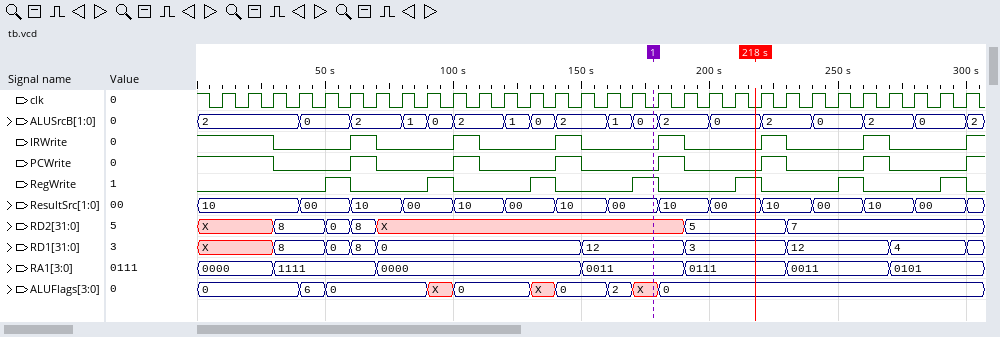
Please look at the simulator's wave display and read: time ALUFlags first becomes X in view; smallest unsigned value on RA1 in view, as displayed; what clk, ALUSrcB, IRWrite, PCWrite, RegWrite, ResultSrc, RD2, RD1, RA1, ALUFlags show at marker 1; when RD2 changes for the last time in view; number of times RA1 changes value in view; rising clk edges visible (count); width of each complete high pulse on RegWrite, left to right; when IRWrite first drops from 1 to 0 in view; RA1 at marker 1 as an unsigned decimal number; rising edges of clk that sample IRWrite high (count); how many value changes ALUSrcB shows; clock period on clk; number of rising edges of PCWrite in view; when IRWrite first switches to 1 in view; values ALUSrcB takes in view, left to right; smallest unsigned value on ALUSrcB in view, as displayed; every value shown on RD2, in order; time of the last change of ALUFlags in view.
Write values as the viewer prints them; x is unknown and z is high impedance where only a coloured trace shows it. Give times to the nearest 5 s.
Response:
90 s
0000
clk=0, ALUSrcB=0, IRWrite=0, PCWrite=0, RegWrite=1, ResultSrc=00, RD2=X, RD1=12, RA1=0011, ALUFlags=X
230 s
6
30
10 s, 10 s, 10 s, 10 s, 10 s, 10 s, 10 s
30 s
3
9
17
10 s
7
60 s
2, 0, 2, 1, 0, 2, 1, 0, 2, 1, 0, 2, 0, 2, 0, 2, 0, 2
0
X, 8, 0, 8, X, 5, 7
180 s
